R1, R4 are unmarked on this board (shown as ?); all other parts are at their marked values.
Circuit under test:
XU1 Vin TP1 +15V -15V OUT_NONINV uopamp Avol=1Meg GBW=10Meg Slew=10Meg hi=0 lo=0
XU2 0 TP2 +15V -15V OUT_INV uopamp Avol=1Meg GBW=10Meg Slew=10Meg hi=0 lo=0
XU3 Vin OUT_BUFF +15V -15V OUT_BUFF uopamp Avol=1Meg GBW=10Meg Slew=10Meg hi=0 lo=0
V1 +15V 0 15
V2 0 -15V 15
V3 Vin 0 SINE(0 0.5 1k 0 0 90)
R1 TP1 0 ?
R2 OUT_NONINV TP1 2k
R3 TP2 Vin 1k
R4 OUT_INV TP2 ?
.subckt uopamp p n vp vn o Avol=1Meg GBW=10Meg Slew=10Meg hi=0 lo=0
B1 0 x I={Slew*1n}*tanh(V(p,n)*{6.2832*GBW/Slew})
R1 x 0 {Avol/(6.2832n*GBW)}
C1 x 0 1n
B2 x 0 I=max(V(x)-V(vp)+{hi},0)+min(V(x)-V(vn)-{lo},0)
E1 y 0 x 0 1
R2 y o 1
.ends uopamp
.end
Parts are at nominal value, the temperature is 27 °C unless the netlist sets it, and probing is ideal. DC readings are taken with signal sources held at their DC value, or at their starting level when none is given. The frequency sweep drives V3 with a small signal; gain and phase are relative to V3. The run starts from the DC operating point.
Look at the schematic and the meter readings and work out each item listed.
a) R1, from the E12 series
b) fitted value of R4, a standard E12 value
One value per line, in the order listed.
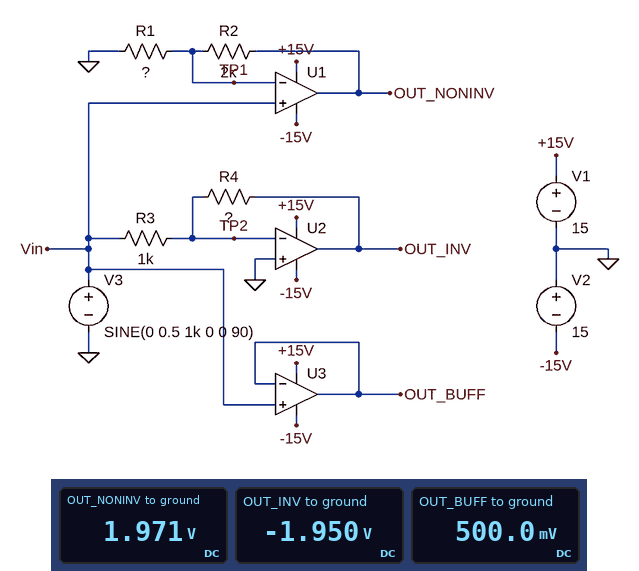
680 Ω
3.9 kΩ
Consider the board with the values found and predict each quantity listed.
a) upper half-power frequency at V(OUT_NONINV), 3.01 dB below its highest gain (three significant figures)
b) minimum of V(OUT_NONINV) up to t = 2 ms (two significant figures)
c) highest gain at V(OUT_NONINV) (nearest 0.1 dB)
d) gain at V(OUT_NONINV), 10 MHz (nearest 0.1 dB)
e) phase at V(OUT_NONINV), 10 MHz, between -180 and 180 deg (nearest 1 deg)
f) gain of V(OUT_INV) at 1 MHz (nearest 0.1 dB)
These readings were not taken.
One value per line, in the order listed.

2.54 MHz
-2.0 V
11.9 dB
-0.3 dB
-76 deg
10.9 dB
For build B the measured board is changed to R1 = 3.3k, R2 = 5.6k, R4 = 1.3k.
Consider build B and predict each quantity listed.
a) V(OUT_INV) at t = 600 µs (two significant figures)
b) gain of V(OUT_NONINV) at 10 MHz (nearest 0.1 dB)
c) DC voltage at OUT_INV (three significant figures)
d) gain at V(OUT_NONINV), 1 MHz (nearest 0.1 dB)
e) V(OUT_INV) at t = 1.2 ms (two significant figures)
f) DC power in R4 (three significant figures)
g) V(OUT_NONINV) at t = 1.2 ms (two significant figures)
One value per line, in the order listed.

530 mV
-0.6 dB
-650 mV
8.3 dB
-200 mV
325 µW
420 mV
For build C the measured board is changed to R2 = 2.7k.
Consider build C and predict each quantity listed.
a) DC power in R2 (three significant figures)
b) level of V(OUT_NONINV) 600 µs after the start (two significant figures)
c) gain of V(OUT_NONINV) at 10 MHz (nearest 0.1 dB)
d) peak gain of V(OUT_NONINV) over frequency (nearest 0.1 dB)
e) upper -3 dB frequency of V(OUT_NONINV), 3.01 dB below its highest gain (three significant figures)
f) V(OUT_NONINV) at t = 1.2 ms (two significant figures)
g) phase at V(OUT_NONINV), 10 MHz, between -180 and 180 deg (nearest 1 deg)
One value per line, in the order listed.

1.46 mW
-2.0 V
-0.2 dB
13.9 dB
2.01 MHz
770 mV
-79 deg
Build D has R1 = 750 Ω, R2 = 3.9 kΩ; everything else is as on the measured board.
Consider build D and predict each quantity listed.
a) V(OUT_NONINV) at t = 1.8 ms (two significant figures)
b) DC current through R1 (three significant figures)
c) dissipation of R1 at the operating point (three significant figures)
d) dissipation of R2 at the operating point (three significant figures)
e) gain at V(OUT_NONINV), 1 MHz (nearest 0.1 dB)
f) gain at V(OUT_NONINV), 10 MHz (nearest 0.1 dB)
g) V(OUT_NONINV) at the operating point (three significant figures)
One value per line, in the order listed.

960 mV
667 µA
333 µW
1.73 mW
14.4 dB
-0.1 dB
3.10 V
